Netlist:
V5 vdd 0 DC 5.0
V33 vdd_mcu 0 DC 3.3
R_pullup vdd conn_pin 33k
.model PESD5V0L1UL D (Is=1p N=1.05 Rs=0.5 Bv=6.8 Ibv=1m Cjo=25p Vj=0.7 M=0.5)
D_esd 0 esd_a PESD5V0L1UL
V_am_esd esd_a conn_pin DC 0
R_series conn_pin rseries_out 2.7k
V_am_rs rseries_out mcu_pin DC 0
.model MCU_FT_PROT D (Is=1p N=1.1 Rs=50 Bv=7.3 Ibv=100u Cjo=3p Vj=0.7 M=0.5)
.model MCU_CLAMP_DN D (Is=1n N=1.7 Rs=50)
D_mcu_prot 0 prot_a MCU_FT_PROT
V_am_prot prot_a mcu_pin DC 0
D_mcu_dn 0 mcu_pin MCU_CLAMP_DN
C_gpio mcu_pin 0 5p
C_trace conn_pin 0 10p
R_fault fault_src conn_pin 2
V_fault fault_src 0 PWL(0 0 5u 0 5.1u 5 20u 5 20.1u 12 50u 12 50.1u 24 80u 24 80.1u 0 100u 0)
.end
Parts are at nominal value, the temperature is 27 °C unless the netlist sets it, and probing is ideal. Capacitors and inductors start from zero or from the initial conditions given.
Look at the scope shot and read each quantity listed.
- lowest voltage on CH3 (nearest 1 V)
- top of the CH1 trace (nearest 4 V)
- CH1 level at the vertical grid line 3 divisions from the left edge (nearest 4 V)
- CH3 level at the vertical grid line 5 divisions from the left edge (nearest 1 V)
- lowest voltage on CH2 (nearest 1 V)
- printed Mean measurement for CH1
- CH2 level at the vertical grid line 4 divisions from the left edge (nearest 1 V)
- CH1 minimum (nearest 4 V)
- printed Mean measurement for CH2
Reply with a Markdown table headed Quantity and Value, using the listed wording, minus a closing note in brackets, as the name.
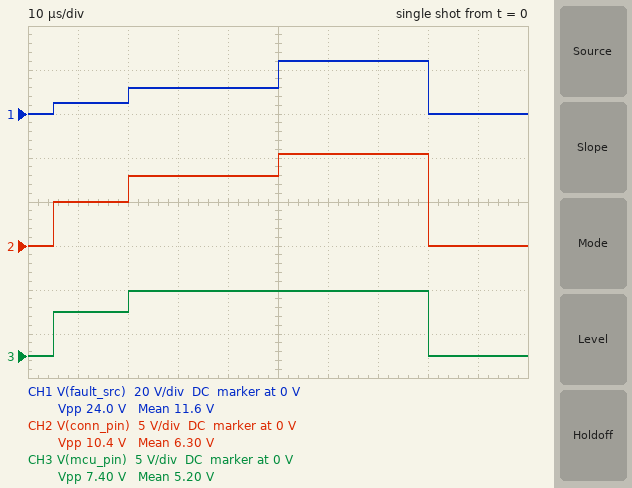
| Quantity | Value |
|---|---|
| lowest voltage on CH3 | 0 V |
| top of the CH1 trace | 24 V |
| CH1 level at the vertical grid line 3 divisions from the left edge | 12 V |
| CH3 level at the vertical grid line 5 divisions from the left edge | 7 V |
| lowest voltage on CH2 | 0 V |
| printed Mean measurement for CH1 | 11.6 V |
| CH2 level at the vertical grid line 4 divisions from the left edge | 8 V |
| CH1 minimum | 0 V |
| printed Mean measurement for CH2 | 6.30 V |
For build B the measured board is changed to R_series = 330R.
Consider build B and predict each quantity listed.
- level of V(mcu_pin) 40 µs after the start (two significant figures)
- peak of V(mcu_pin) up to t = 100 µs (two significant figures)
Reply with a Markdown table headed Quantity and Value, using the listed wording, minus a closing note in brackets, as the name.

| Quantity | Value |
|---|---|
| level of V(mcu_pin) 40 µs after the start | 7.5 V |
| peak of V(mcu_pin) up to t = 100 µs | 7.8 V |
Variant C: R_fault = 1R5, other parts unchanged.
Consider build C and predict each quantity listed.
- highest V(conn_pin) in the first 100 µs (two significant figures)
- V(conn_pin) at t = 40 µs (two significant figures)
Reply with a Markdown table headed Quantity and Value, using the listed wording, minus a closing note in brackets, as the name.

| Quantity | Value |
|---|---|
| highest V(conn_pin) in the first 100 µs | 11 V |
| V(conn_pin) at t = 40 µs | 8.3 V |
